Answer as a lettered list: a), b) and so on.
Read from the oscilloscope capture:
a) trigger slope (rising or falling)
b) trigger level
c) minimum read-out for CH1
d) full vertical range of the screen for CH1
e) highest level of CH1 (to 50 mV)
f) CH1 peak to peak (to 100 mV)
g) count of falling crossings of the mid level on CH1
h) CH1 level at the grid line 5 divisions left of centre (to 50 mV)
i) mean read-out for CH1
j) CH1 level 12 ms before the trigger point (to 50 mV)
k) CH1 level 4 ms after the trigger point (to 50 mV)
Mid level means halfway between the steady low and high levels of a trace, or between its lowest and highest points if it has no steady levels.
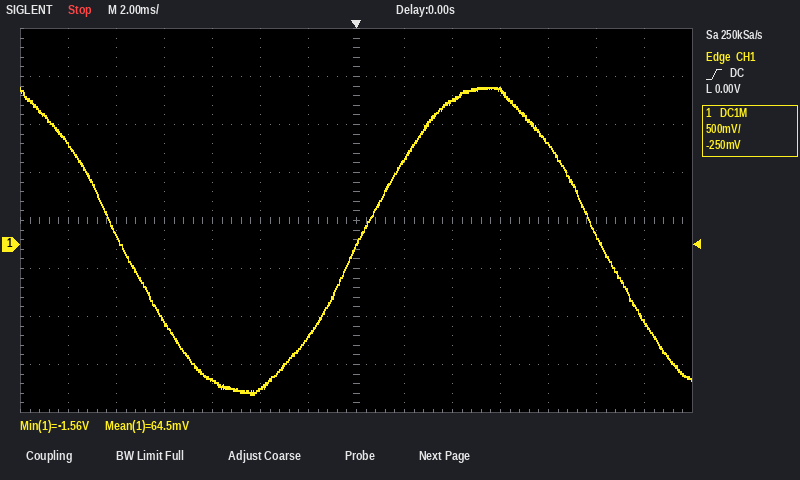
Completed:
a) rising
b) 0.00 V
c) -1.56 V
d) 4 V
e) 1.65 V
f) 3.20 V
g) 2
h) 100 mV
i) 64.5 mV
j) 1.05 V
k) 1.50 V
